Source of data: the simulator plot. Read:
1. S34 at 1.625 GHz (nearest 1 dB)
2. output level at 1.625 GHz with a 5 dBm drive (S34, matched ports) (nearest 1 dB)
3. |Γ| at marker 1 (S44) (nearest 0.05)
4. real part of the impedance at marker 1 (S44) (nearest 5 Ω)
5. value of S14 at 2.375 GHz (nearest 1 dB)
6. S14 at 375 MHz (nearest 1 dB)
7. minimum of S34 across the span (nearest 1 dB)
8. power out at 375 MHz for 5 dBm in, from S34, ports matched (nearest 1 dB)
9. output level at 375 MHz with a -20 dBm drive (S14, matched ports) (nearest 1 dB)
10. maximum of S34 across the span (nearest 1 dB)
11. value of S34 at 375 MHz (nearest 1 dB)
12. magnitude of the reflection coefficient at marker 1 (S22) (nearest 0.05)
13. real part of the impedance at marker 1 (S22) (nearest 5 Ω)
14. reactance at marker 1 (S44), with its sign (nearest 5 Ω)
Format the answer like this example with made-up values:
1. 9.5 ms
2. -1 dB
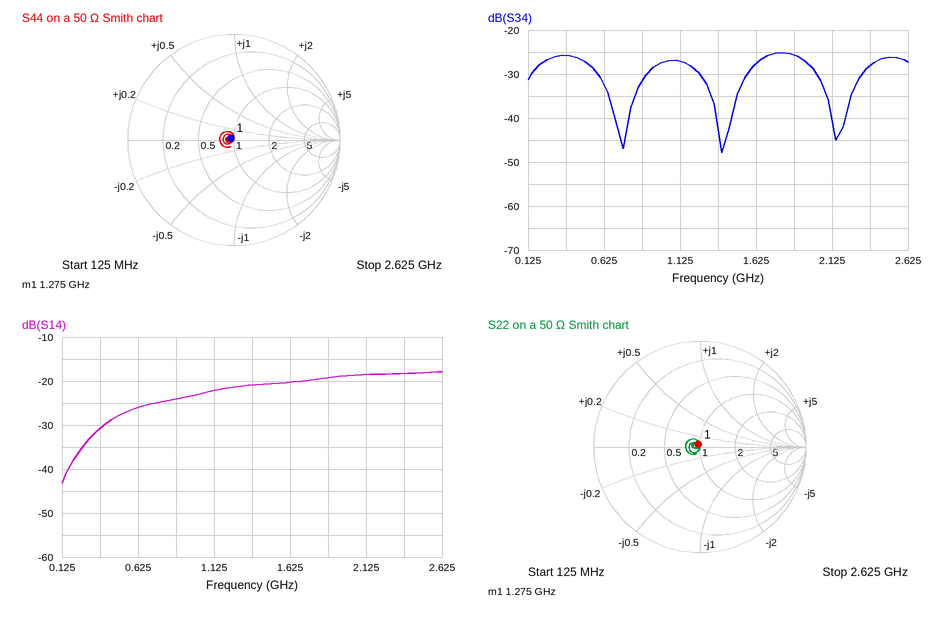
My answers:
1. -28 dB
2. -23 dBm
3. 0.05
4. 45 Ω
5. -18 dB
6. -31 dB
7. -48 dB
8. -21 dBm
9. -51 dBm
10. -25 dB
11. -26 dB
12. 0.05
13. 50 Ω
14. 0 Ω
